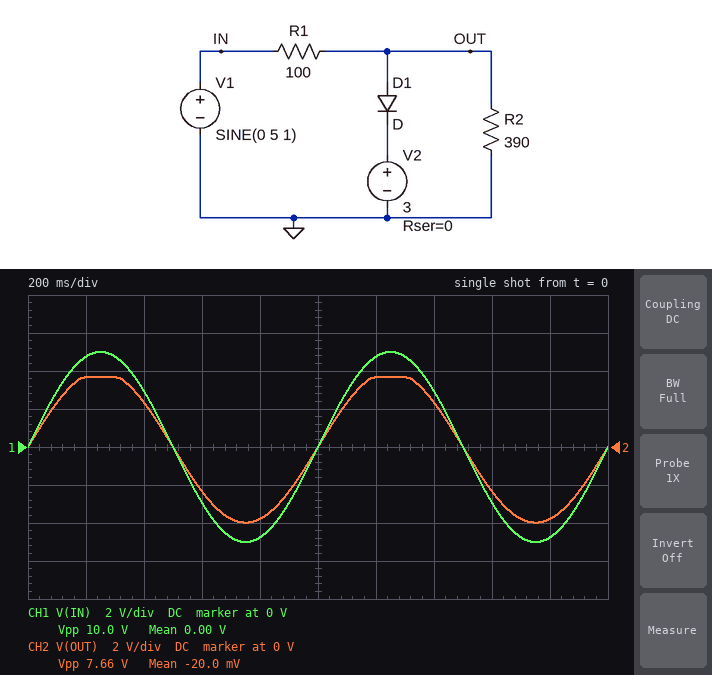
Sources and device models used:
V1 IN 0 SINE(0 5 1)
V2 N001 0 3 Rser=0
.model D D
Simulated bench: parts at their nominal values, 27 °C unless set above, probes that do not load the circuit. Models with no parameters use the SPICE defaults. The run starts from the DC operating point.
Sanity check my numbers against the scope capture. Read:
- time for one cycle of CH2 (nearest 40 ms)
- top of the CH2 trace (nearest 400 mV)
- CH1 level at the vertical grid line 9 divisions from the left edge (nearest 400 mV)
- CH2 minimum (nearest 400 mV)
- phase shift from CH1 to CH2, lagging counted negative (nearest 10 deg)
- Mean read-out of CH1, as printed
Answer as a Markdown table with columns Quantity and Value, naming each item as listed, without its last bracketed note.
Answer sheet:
| Quantity | Value |
|---|---|
| time for one cycle of CH2 | 1.00 s |
| top of the CH2 trace | 3.6 V |
| CH1 level at the vertical grid line 9 divisions from the left edge | -4.8 V |
| CH2 minimum | -4.0 V |
| phase shift from CH1 to CH2, lagging counted negative | 0 deg |
| Mean read-out of CH1, as printed | 0.00 V |
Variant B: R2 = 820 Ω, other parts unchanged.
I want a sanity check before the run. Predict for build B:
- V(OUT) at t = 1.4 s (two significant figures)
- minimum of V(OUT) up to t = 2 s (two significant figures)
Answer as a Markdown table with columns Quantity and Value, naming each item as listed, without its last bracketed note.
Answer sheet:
| Quantity | Value |
|---|---|
| V(OUT) at t = 1.4 s | 2.6 V |
| minimum of V(OUT) up to t = 2 s | -4.5 V |
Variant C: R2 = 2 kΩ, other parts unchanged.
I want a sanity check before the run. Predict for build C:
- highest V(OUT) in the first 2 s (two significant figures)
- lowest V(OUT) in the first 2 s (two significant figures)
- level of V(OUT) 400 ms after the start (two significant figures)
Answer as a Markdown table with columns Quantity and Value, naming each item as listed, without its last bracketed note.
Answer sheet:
| Quantity | Value |
|---|---|
| highest V(OUT) in the first 2 s | 3.7 V |
| lowest V(OUT) in the first 2 s | -4.8 V |
| level of V(OUT) 400 ms after the start | 2.8 V |
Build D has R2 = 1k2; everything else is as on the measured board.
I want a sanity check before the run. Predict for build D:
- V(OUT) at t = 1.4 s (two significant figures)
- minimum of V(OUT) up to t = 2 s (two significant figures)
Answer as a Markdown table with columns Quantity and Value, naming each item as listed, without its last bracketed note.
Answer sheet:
| Quantity | Value |
|---|---|
| V(OUT) at t = 1.4 s | 2.7 V |
| minimum of V(OUT) up to t = 2 s | -4.6 V |
